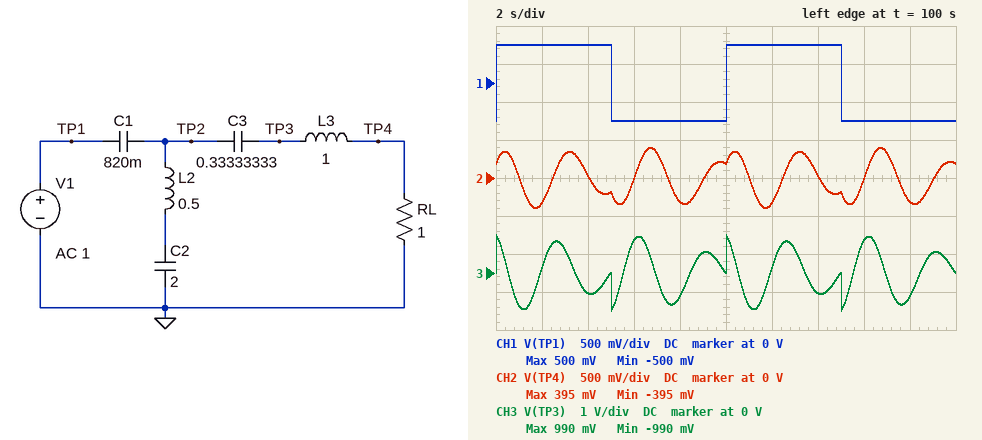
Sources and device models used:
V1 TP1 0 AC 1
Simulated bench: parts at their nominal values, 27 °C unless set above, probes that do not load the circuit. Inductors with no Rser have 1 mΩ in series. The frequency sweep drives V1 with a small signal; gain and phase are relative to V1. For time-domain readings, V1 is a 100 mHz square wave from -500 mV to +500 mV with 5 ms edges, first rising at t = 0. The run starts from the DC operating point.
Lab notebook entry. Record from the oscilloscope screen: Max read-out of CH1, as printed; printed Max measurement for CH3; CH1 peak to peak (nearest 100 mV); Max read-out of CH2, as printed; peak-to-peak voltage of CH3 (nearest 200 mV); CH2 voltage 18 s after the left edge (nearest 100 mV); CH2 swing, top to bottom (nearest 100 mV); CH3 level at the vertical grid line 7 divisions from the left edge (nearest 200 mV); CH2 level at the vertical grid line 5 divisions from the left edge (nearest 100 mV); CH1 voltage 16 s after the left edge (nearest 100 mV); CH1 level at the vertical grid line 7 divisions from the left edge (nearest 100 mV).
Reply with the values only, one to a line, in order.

500 mV
990 mV
1.0 V
395 mV
2.0 V
-300 mV
800 mV
-600 mV
200 mV
-500 mV
500 mV
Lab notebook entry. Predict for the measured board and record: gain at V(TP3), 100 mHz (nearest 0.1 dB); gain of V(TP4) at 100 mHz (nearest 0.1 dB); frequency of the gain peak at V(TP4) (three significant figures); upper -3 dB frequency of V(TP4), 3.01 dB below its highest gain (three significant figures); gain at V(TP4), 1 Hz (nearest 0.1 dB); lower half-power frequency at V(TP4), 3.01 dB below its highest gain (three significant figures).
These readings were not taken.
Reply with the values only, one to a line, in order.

-25.9 dB
-27.4 dB
358 mHz
405 mHz
-14.5 dB
304 mHz
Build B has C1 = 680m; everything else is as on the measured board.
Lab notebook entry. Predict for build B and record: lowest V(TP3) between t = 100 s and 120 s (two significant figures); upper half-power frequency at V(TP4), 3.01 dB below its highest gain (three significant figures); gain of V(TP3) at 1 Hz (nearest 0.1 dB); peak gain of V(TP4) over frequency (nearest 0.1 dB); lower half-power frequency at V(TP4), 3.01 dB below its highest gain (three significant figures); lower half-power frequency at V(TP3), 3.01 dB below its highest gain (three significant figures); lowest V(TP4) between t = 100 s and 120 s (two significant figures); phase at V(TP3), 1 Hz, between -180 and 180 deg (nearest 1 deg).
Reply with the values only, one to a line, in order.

-810 mV
427 mHz
1.7 dB
7.5 dB
339 mHz
347 mHz
-330 mV
1 deg
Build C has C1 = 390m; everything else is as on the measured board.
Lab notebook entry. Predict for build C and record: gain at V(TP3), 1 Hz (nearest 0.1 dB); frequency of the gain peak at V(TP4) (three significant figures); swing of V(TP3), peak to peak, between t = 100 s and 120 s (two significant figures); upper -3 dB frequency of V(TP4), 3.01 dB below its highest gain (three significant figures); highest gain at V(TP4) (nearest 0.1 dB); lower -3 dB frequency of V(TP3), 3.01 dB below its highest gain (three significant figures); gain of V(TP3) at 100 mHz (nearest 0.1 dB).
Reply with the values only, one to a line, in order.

2.6 dB
481 mHz
2.8 V
517 mHz
8.3 dB
450 mHz
-31.5 dB
